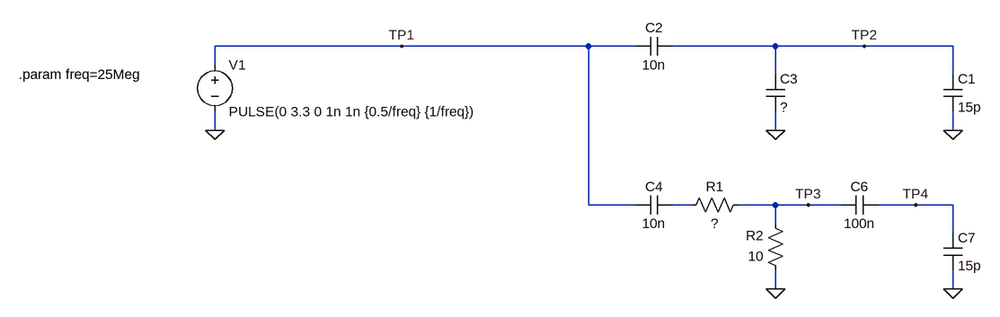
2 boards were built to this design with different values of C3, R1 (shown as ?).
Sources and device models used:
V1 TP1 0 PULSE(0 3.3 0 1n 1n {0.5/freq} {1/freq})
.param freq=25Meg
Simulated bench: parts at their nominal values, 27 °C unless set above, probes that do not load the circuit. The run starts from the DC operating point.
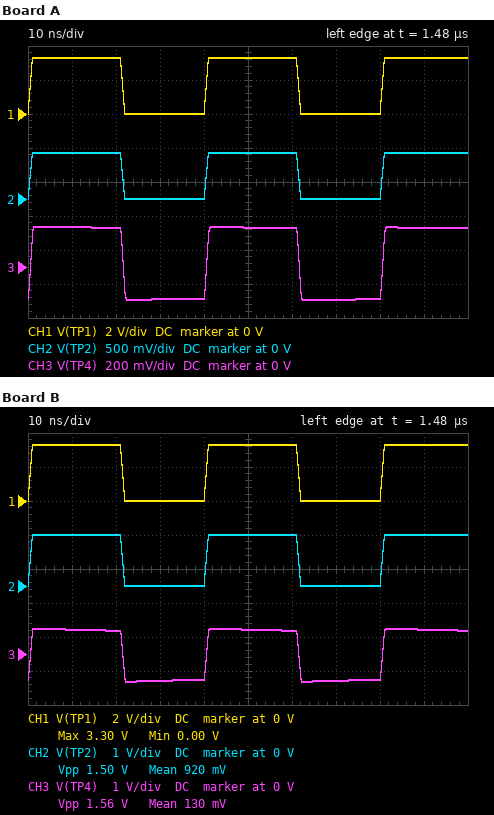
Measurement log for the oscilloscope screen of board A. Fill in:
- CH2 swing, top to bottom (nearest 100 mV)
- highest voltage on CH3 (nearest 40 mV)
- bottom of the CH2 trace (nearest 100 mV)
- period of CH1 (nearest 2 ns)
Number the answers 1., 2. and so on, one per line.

1. 700 mV
2. 240 mV
3. 0 V
4. 40 ns
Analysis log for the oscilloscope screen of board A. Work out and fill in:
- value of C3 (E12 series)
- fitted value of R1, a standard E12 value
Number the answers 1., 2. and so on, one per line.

1. 39 nF
2. 68 Ω
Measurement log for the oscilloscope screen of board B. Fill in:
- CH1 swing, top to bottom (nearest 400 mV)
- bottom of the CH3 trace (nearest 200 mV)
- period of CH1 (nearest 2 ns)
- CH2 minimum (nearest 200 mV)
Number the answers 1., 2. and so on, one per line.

1. 3.2 V
2. -800 mV
3. 40 ns
4. 0 V
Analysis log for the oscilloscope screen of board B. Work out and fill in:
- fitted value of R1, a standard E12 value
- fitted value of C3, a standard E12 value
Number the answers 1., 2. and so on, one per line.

1. 12 Ω
2. 12 nF
